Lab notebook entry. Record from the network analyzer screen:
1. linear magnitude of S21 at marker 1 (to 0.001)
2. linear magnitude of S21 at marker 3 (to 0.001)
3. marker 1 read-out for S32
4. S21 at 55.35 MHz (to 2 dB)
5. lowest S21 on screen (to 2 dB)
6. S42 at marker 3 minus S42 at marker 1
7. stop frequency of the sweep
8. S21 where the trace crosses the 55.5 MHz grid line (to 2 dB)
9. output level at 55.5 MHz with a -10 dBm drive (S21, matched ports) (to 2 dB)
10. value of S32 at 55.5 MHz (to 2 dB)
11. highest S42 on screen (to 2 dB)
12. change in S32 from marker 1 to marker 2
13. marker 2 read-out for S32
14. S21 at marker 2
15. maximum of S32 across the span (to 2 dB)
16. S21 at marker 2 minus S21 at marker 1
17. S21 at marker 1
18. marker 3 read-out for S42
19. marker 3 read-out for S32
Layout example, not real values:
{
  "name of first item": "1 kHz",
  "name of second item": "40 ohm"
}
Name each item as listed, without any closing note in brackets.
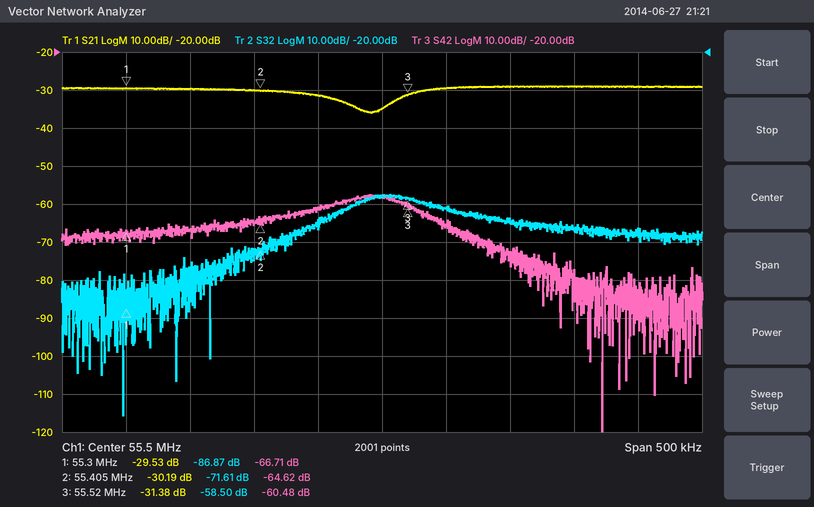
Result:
{
  "linear magnitude of S21 at marker 1": "0.033",
  "linear magnitude of S21 at marker 3": "0.027",
  "marker 1 read-out for S32": "-86.87 dB",
  "S21 at 55.35 MHz": "-30 dB",
  "lowest S21 on screen": "-36 dB",
  "S42 at marker 3 minus S42 at marker 1": "6.23 dB",
  "stop frequency of the sweep": "55.75 MHz",
  "S21 where the trace crosses the 55.5 MHz grid line": "-34 dB",
  "output level at 55.5 MHz with a -10 dBm drive (S21, matched ports)": "-44 dBm",
  "value of S32 at 55.5 MHz": "-58 dB",
  "highest S42 on screen": "-58 dB",
  "change in S32 from marker 1 to marker 2": "15.26 dB",
  "marker 2 read-out for S32": "-71.61 dB",
  "S21 at marker 2": "-30.19 dB",
  "maximum of S32 across the span": "-58 dB",
  "S21 at marker 2 minus S21 at marker 1": "-0.66 dB",
  "S21 at marker 1": "-29.53 dB",
  "marker 3 read-out for S42": "-60.48 dB",
  "marker 3 read-out for S32": "-58.50 dB"
}
